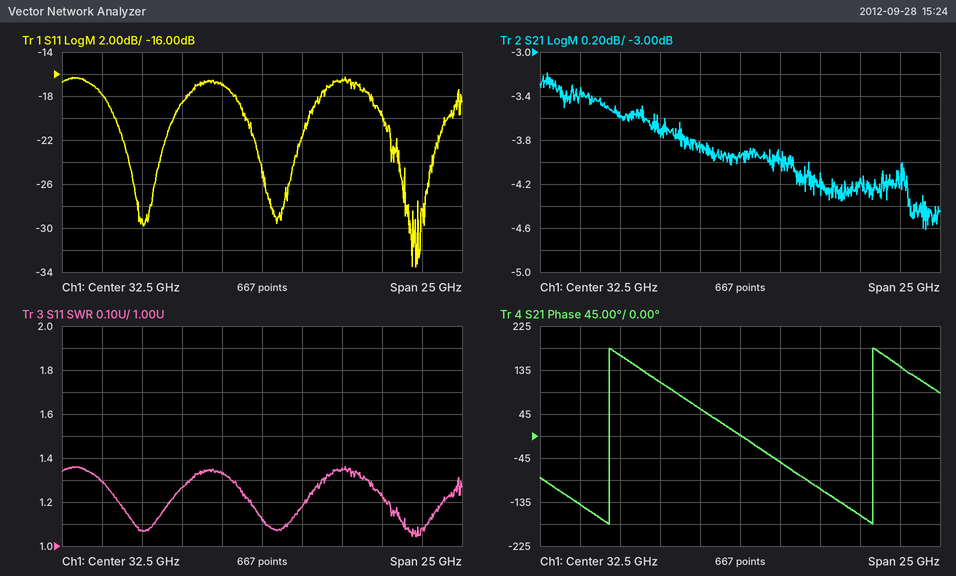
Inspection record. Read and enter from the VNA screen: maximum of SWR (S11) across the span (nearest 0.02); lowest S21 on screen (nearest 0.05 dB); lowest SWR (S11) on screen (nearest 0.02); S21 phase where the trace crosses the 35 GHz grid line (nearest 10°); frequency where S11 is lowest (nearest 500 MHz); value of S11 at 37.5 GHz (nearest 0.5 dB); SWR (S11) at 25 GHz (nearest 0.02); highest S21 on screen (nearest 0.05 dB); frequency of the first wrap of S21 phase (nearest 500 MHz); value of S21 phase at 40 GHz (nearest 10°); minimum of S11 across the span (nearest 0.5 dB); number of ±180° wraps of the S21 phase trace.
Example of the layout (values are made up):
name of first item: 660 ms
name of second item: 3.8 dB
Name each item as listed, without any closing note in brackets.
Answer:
maximum of SWR (S11) across the span: 1.36
lowest S21 on screen: -4.60 dB
lowest SWR (S11) on screen: 1.04
S21 phase where the trace crosses the 35 GHz grid line: -50°
frequency where S11 is lowest: 42.0 GHz
value of S11 at 37.5 GHz: -16.5 dB
SWR (S11) at 25 GHz: 1.08
highest S21 on screen: -3.20 dB
frequency of the first wrap of S21 phase: 24.5 GHz
value of S21 phase at 40 GHz: -160°
minimum of S11 across the span: -33.5 dB
number of ±180° wraps of the S21 phase trace: 2
